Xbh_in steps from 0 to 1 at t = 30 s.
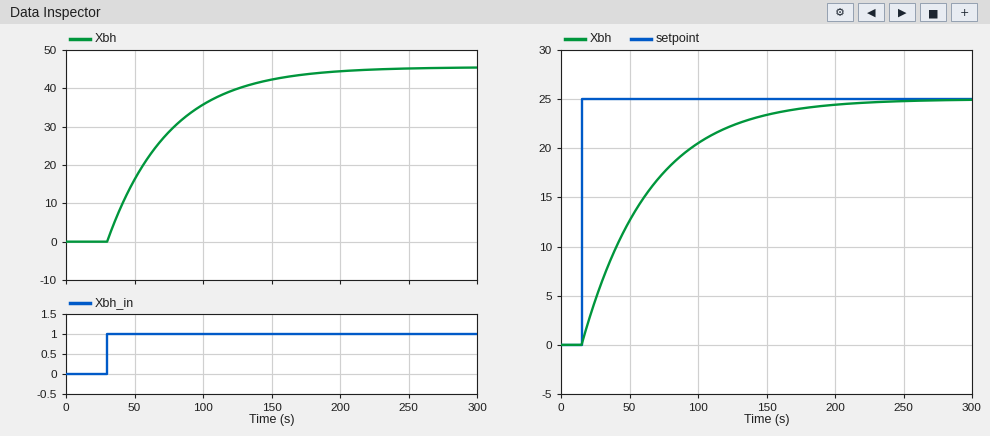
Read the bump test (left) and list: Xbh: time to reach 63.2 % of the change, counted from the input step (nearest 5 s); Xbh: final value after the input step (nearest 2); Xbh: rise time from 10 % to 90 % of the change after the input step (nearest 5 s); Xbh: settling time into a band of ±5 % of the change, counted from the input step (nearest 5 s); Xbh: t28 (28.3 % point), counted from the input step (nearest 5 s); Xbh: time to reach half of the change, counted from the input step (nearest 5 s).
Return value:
45 s
46
100 s
135 s
15 s
30 s
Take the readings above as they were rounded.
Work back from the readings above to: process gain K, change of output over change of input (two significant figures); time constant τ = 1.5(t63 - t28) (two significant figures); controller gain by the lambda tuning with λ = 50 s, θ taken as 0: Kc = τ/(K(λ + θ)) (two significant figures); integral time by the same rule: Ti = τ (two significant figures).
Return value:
46
45 s
0.020
45 s
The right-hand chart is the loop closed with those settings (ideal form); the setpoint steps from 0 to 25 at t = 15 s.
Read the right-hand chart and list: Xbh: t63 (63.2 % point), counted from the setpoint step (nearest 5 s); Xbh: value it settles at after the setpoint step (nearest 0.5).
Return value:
50 s
25.0
